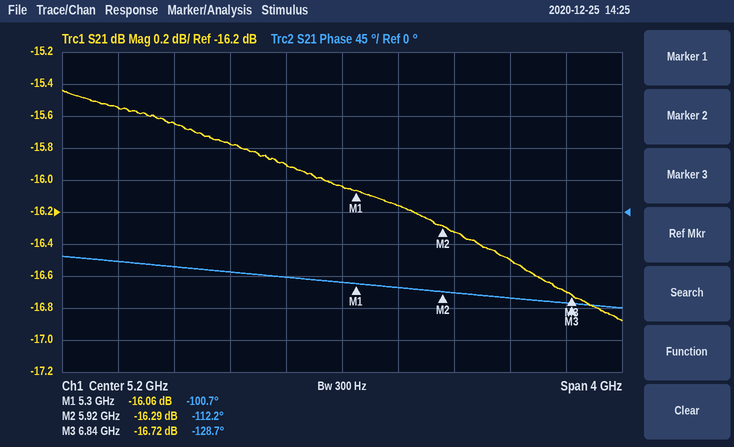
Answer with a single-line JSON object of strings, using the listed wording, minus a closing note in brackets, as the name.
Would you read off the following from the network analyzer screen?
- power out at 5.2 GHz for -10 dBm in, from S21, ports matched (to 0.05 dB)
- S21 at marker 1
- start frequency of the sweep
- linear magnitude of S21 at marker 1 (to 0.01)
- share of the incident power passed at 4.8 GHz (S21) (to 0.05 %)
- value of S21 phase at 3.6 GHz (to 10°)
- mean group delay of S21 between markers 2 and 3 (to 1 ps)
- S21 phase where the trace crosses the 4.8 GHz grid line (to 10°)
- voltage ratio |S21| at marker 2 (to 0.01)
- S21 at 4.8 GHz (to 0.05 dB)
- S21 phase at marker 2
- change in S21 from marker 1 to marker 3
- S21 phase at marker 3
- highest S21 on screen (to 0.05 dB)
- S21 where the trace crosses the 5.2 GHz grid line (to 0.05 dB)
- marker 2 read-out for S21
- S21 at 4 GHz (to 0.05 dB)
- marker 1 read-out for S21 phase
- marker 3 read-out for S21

{"power out at 5.2 GHz for -10 dBm in, from S21, ports matched": "-26.05 dBm", "S21 at marker 1": "-16.06 dB", "start frequency of the sweep": "3.2 GHz", "linear magnitude of S21 at marker 1": "0.16", "share of the incident power passed at 4.8 GHz (S21)": "2.55 %", "value of S21 phase at 3.6 GHz": "-70°", "mean group delay of S21 between markers 2 and 3": "50 ps", "S21 phase where the trace crosses the 4.8 GHz grid line": "-90°", "voltage ratio |S21| at marker 2": "0.15", "S21 at 4.8 GHz": "-15.90 dB", "S21 phase at marker 2": "-112.2°", "change in S21 from marker 1 to marker 3": "-0.66 dB", "S21 phase at marker 3": "-128.7°", "highest S21 on screen": "-15.45 dB", "S21 where the trace crosses the 5.2 GHz grid line": "-16.05 dB", "marker 2 read-out for S21": "-16.29 dB", "S21 at 4 GHz": "-15.65 dB", "marker 1 read-out for S21 phase": "-100.7°", "marker 3 read-out for S21": "-16.72 dB"}
